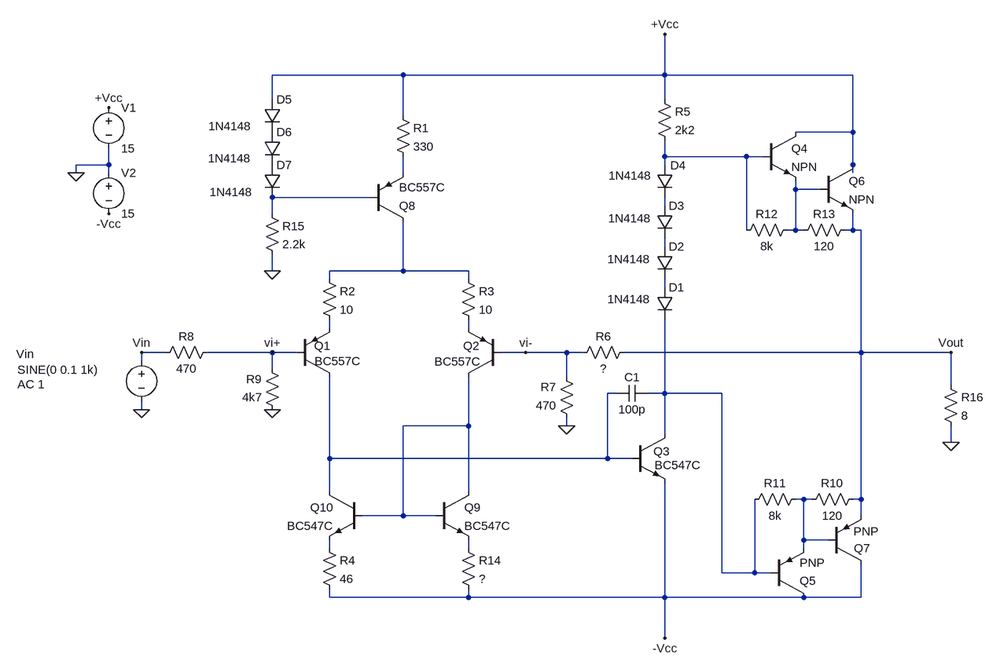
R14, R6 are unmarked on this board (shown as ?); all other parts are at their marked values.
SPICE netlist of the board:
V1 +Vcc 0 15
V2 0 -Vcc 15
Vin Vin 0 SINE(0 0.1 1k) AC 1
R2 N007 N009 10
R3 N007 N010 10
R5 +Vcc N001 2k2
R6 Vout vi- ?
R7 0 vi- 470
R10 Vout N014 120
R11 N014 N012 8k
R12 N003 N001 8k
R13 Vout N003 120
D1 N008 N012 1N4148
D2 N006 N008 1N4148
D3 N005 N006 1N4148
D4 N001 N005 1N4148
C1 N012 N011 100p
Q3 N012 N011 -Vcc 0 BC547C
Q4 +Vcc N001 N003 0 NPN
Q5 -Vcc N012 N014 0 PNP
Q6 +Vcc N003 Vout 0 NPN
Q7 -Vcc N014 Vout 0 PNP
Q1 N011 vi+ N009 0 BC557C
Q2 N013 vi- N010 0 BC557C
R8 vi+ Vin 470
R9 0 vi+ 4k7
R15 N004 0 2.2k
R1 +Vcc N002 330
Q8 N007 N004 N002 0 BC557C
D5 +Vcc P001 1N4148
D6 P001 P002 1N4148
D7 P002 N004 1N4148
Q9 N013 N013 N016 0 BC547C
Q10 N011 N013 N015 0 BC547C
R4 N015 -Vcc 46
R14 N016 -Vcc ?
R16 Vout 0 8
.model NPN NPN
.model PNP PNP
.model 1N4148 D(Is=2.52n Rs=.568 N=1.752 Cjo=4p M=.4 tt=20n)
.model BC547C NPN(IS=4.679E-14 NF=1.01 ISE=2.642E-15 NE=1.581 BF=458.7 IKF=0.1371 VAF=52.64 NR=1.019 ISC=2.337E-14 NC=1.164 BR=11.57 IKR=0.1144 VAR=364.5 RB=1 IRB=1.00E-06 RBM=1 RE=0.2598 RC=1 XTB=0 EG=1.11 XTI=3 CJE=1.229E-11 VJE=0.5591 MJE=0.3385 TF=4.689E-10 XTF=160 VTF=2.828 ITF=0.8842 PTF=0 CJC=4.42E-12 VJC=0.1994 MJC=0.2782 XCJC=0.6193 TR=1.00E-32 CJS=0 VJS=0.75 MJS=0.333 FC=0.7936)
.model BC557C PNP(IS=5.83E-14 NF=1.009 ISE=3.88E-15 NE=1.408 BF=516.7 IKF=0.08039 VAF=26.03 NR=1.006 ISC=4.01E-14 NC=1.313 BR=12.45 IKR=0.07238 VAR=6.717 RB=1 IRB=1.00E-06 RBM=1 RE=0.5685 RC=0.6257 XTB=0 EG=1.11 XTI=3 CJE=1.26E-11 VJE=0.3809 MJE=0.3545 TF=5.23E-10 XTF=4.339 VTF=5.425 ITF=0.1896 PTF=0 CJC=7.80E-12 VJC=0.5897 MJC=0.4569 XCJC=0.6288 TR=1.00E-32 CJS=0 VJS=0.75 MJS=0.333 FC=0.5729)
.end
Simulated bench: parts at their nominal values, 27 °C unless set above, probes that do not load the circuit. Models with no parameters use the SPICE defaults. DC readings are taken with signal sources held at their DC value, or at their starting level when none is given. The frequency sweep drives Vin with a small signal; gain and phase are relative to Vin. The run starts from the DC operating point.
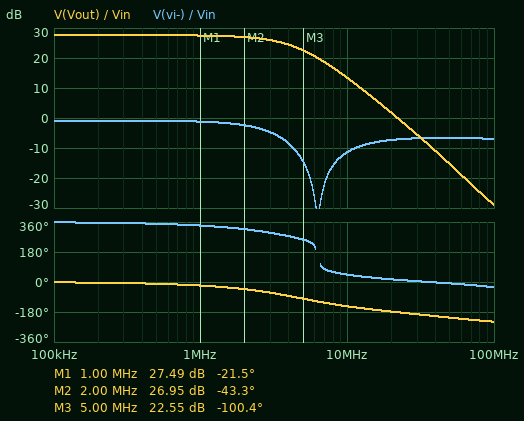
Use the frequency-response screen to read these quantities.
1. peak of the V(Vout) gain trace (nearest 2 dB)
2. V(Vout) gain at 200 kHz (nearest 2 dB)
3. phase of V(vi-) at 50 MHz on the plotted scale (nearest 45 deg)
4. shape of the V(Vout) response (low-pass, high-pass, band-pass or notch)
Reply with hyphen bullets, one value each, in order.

- 28 dB
- 28 dB
- 0 deg
- low-pass
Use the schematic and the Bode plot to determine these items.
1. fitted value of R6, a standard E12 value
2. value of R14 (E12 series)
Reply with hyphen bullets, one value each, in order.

- 12 kΩ
- 68 Ω
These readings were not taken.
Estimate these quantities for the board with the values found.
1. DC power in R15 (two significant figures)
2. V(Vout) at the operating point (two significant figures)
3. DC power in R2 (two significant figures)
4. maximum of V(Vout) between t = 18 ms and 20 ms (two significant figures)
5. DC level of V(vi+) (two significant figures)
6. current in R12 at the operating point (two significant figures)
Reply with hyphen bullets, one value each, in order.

- 77 mW
- 410 mV
- 56 µW
- 2.8 V
- 1.4 mV
- 100 µA
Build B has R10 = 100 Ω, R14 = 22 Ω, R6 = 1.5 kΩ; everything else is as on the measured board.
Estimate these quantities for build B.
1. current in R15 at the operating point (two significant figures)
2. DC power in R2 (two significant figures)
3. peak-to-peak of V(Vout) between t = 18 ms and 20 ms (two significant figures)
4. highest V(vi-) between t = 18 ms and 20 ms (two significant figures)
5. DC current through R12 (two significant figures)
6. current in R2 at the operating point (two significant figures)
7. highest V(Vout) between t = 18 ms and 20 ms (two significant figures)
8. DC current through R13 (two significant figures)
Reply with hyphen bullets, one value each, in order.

- 5.9 mA
- 24 µW
- 760 mV
- 67 mV
- 99 µA
- 1.5 mA
- 280 mV
- 2.0 mA
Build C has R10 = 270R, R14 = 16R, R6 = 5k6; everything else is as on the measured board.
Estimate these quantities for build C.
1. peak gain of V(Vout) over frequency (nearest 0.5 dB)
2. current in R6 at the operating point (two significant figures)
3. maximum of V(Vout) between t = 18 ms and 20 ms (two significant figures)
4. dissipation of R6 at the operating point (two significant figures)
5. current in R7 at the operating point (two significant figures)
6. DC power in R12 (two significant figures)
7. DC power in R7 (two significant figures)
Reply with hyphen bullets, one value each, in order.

- 21.5 dB
- 72 µA
- 740 mV
- 29 µW
- 68 µA
- 78 µW
- 2.2 µW
